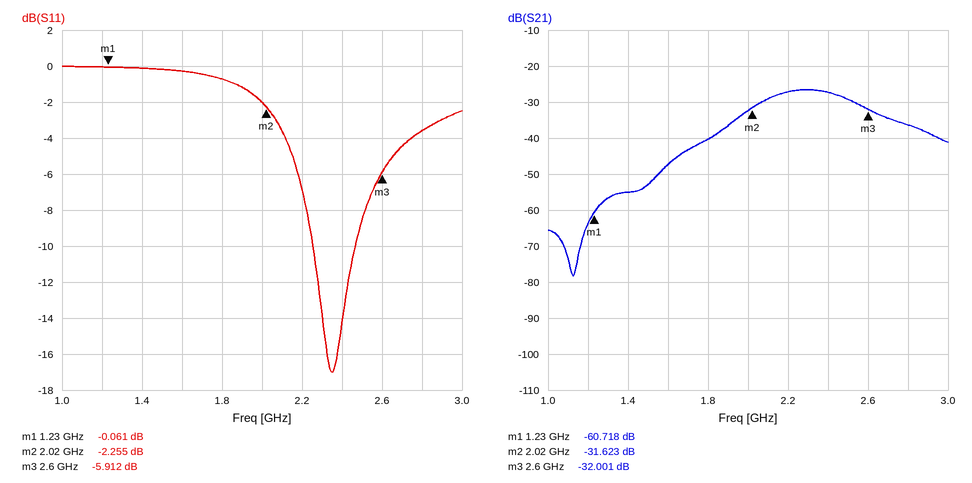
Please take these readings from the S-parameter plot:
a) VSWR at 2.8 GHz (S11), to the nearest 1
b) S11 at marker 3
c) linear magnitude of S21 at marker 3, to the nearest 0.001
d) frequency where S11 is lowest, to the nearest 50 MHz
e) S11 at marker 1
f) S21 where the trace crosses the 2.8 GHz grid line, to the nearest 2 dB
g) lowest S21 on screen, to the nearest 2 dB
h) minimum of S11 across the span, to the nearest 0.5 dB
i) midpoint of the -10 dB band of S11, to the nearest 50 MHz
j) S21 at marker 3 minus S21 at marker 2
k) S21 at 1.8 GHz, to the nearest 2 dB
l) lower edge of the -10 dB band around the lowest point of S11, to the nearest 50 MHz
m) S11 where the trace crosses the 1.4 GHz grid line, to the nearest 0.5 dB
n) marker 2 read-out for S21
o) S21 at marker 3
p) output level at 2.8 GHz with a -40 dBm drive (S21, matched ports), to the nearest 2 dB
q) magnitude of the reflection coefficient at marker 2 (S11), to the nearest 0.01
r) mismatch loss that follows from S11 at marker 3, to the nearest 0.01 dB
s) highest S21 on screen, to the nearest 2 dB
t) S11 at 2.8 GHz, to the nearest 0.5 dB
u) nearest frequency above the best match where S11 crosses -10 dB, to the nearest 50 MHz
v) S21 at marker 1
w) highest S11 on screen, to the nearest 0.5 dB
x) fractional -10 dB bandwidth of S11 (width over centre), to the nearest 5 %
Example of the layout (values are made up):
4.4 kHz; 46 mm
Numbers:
5; -5.912 dB; 0.025; 2.35 GHz; -0.061 dB; -36 dB; -78 dB; -17.0 dB; 2.35 GHz; -0.378 dB; -40 dB; 2.25 GHz; 0.0 dB; -31.623 dB; -32.001 dB; -76 dBm; 0.77; 1.29 dB; -26 dB; -3.5 dB; 2.45 GHz; -60.718 dB; 0.0 dB; 10 %
